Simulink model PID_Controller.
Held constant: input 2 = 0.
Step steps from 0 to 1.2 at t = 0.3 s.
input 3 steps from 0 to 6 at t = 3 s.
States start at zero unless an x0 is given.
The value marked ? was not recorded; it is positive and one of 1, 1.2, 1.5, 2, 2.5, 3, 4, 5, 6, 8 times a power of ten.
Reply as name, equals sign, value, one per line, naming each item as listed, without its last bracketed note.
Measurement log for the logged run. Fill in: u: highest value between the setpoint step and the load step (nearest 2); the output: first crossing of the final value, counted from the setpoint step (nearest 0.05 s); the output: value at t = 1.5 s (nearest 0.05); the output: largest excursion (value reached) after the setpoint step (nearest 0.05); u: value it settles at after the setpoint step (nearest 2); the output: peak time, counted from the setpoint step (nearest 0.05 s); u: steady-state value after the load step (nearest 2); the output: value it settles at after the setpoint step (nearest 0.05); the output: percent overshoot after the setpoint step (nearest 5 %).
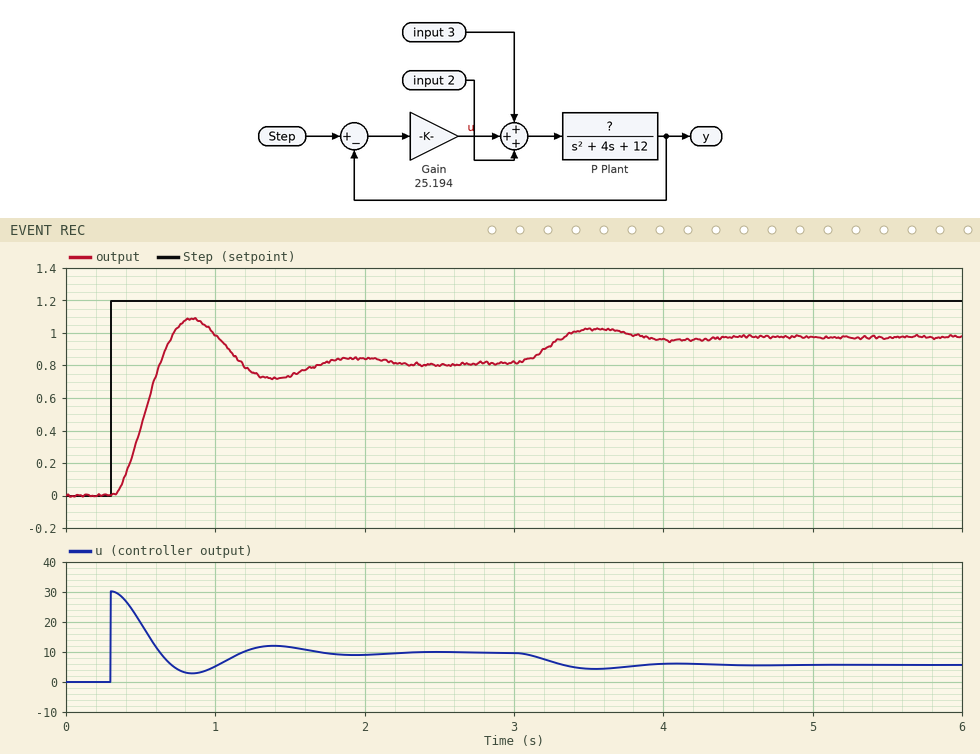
u: highest value between the setpoint step and the load step = 30
the output: first crossing of the final value, counted from the setpoint step = 0.35 s
the output: value at t = 1.5 s = 0.75
the output: largest excursion (value reached) after the setpoint step = 1.10
u: value it settles at after the setpoint step = 10
the output: peak time, counted from the setpoint step = 0.55 s
u: steady-state value after the load step = 6
the output: value it settles at after the setpoint step = 0.80
the output: percent overshoot after the setpoint step = 35 %
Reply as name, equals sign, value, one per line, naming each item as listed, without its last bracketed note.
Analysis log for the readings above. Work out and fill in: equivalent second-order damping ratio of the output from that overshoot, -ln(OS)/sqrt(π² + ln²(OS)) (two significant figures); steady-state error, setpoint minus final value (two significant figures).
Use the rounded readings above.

equivalent second-order damping ratio of the output from that overshoot, -ln(OS)/sqrt(π² + ln²(OS)) = 0.32
steady-state error, setpoint minus final value = 0.40
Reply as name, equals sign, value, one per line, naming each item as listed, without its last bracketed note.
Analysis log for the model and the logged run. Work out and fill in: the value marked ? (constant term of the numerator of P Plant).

the value marked ? = 1
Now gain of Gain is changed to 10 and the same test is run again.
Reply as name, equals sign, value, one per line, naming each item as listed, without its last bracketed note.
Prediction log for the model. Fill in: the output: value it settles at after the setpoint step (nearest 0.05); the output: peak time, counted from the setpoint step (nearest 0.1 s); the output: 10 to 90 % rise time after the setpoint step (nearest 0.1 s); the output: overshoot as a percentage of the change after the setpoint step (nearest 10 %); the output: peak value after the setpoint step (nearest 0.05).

the output: value it settles at after the setpoint step = 0.55
the output: peak time, counted from the setpoint step = 0.7 s
the output: 10 to 90 % rise time after the setpoint step = 0.3 s
the output: overshoot as a percentage of the change after the setpoint step = 20 %
the output: peak value after the setpoint step = 0.65
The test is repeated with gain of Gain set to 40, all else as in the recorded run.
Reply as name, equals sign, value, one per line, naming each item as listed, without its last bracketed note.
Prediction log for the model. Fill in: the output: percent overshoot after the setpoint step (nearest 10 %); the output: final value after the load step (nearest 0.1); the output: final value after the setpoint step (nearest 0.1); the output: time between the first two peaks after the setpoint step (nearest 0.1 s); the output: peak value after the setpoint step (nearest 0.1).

the output: percent overshoot after the setpoint step = 40 %
the output: final value after the load step = 1.0
the output: final value after the setpoint step = 0.9
the output: time between the first two peaks after the setpoint step = 0.9 s
the output: peak value after the setpoint step = 1.3
